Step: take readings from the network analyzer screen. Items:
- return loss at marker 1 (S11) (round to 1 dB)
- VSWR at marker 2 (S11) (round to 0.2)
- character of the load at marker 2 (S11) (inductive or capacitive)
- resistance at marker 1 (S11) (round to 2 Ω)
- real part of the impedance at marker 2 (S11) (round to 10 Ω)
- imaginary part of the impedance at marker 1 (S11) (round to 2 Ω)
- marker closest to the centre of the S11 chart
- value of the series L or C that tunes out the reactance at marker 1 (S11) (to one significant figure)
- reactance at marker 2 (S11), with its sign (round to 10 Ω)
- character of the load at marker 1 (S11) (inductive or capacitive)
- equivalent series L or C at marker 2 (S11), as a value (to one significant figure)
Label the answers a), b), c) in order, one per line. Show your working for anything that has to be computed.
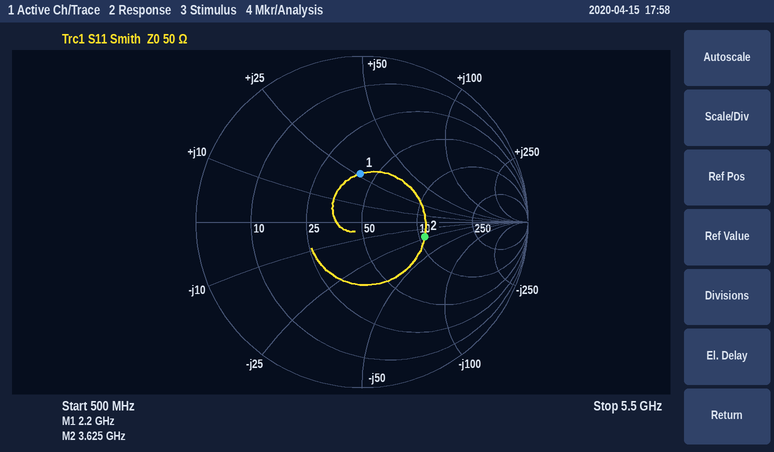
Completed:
a) 11 dB
b) 2.2
c) capacitive
d) 42 Ω
e) 110 Ω
f) +26 Ω
g) marker 1
h) C = 1/(2π × 2.2 GHz × 26 Ω) ≈ 3 pF
i) -20 Ω
j) inductive
k) C = 1/(2π × 3.625 GHz × 20 Ω) ≈ 2 pF
